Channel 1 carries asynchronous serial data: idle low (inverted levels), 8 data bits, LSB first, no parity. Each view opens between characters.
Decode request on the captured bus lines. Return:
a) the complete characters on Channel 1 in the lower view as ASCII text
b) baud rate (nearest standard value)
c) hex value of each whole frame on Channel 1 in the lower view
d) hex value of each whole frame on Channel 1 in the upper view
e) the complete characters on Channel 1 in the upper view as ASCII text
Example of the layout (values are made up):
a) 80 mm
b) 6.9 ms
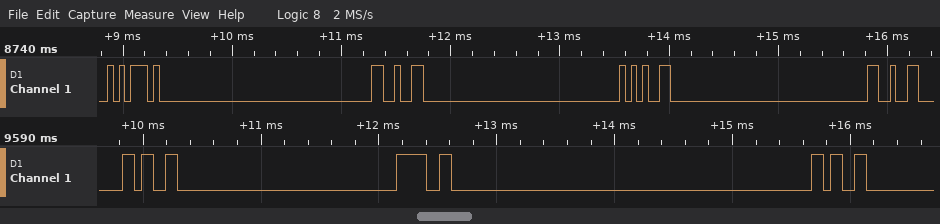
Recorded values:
a) "202"
b) 19200 baud
c) 32, 30, 32
d) 45, 36, 35, 36
e) "E656"
